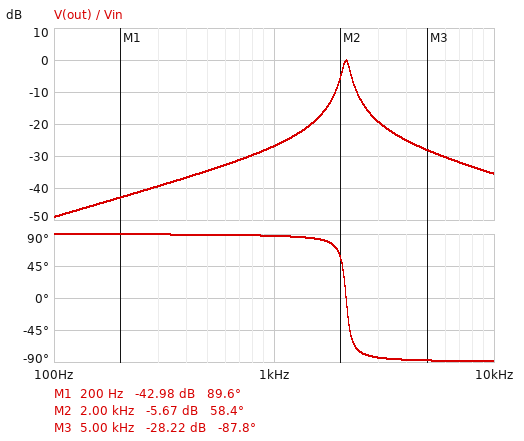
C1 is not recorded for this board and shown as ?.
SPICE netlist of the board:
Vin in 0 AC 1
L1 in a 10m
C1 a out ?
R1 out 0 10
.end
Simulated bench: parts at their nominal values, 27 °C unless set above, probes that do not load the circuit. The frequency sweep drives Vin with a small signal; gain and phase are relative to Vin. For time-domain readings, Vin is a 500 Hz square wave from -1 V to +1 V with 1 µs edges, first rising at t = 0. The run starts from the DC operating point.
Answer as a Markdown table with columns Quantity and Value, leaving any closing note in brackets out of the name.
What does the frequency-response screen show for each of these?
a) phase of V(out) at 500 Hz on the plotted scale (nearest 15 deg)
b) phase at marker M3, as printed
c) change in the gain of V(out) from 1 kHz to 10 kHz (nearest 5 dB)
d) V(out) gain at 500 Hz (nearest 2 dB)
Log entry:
| Quantity | Value |
|---|---|
| phase of V(out) at 500 Hz on the plotted scale | 90 deg |
| phase at marker M3, as printed | -87.8 deg |
| change in the gain of V(out) from 1 kHz to 10 kHz | -10 dB |
| V(out) gain at 500 Hz | -34 dB |
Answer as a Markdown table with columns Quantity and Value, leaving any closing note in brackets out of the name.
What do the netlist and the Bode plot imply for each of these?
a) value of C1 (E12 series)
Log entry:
| Quantity | Value |
|---|---|
| value of C1 | 560 nF |
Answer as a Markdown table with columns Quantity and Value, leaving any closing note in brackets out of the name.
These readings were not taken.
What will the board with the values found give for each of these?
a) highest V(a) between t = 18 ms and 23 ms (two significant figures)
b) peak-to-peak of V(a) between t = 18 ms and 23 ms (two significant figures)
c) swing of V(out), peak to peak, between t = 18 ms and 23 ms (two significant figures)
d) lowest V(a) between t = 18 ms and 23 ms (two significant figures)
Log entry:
| Quantity | Value |
|---|---|
| highest V(a) between t = 18 ms and 23 ms | 2.2 V |
| peak-to-peak of V(a) between t = 18 ms and 23 ms | 4.4 V |
| swing of V(out), peak to peak, between t = 18 ms and 23 ms | 190 mV |
| lowest V(a) between t = 18 ms and 23 ms | -2.2 V |
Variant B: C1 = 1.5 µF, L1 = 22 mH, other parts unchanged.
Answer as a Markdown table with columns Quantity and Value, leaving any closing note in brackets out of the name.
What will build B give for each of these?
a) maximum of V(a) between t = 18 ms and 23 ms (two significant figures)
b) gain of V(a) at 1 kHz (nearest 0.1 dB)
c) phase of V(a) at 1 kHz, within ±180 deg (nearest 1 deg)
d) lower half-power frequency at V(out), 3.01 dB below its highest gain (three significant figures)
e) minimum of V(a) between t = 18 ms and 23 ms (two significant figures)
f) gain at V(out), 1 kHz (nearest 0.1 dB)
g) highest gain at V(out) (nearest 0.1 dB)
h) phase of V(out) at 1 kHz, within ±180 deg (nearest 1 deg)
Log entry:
| Quantity | Value |
|---|---|
| maximum of V(a) between t = 18 ms and 23 ms | 2.1 V |
| gain of V(a) at 1 kHz | 10.0 dB |
| phase of V(a) at 1 kHz, within ±180 deg | -157 deg |
| lower half-power frequency at V(out), 3.01 dB below its highest gain | 841 Hz |
| minimum of V(a) between t = 18 ms and 23 ms | -2.1 V |
| gain at V(out), 1 kHz | -10.5 dB |
| highest gain at V(out) | 0 dB |
| phase of V(out) at 1 kHz, within ±180 deg | -73 deg |
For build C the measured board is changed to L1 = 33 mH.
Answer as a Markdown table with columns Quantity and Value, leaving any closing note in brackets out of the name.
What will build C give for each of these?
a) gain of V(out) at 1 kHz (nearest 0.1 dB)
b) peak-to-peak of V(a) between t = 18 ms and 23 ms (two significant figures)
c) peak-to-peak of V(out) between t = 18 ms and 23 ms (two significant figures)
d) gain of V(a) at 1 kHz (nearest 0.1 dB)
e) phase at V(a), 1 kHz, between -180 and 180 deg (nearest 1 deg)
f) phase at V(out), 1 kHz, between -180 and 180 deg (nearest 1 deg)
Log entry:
| Quantity | Value |
|---|---|
| gain of V(out) at 1 kHz | -17.8 dB |
| peak-to-peak of V(a) between t = 18 ms and 23 ms | 4.4 V |
| peak-to-peak of V(out) between t = 18 ms and 23 ms | 100 mV |
| gain of V(a) at 1 kHz | 11.3 dB |
| phase at V(a), 1 kHz, between -180 and 180 deg | -5 deg |
| phase at V(out), 1 kHz, between -180 and 180 deg | 83 deg |
